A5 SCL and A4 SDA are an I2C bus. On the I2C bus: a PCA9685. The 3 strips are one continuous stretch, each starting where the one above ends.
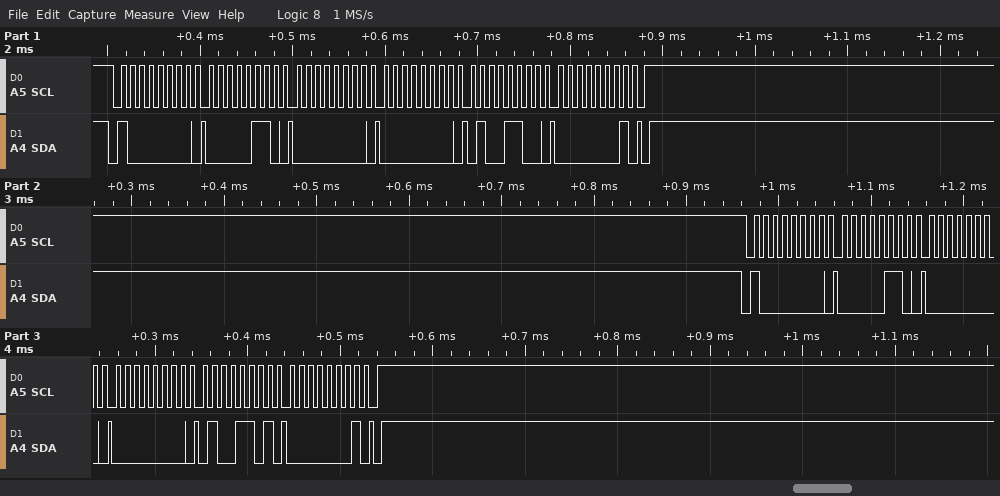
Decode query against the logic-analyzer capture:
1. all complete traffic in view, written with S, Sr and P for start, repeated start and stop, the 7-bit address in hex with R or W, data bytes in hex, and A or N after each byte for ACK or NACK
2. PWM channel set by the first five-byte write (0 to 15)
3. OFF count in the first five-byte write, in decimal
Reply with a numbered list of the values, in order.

1. S 40W A 06 A 00 A 00 A 4C A 01 A P S 40W A 06 A 00 A 00 A 4D A 01 A P
2. 0
3. 332
